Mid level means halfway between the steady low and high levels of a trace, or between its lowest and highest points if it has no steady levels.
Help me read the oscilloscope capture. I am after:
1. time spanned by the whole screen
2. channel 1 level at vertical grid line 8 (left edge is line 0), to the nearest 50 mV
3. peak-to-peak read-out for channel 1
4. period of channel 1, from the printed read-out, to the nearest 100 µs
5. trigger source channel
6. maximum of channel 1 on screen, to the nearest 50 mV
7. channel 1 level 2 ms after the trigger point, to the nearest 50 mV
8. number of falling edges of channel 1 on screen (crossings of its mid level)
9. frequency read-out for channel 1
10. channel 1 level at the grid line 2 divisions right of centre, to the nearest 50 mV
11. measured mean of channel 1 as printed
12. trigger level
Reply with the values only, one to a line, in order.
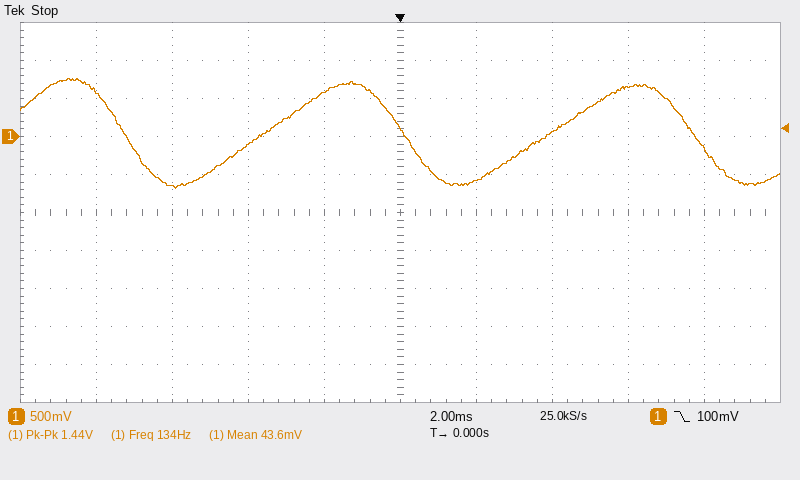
20 ms
650 mV
1.44 V
7.5 ms
channel 1
750 mV
-600 mV
3
134 Hz
50 mV
43.6 mV
100 mV
